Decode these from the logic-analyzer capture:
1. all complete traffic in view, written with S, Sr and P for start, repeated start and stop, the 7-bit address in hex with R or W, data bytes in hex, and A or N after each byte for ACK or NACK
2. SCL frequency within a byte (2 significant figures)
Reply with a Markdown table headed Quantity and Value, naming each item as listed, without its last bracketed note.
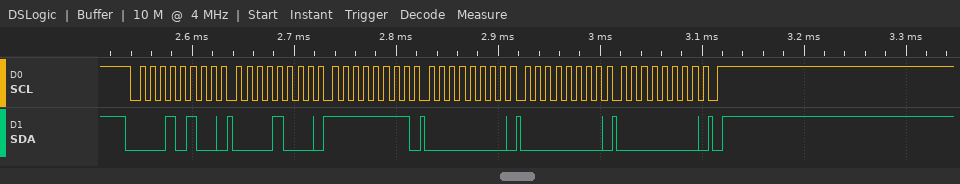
| Quantity | Value |
|---|---|
| all complete traffic in view, written with S, Sr and P for start, repeated start and stop, the 7-bit address in hex with R or W, data bytes in hex, and A or N after each byte for ACK or NACK | S 0AW A 08 A FF A 00 A 00 A 00 A P |
| SCL frequency within a byte | 100 kHz |
